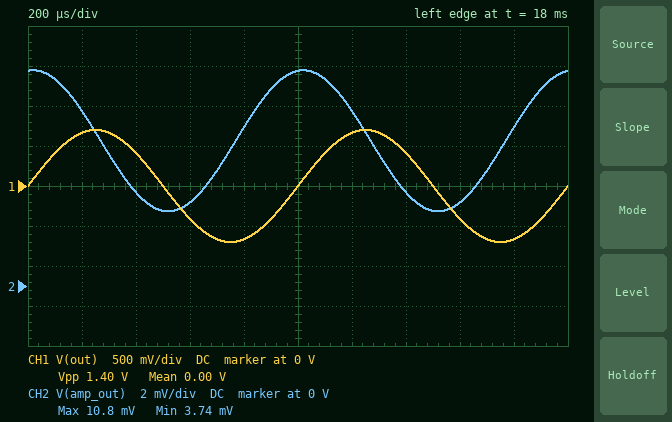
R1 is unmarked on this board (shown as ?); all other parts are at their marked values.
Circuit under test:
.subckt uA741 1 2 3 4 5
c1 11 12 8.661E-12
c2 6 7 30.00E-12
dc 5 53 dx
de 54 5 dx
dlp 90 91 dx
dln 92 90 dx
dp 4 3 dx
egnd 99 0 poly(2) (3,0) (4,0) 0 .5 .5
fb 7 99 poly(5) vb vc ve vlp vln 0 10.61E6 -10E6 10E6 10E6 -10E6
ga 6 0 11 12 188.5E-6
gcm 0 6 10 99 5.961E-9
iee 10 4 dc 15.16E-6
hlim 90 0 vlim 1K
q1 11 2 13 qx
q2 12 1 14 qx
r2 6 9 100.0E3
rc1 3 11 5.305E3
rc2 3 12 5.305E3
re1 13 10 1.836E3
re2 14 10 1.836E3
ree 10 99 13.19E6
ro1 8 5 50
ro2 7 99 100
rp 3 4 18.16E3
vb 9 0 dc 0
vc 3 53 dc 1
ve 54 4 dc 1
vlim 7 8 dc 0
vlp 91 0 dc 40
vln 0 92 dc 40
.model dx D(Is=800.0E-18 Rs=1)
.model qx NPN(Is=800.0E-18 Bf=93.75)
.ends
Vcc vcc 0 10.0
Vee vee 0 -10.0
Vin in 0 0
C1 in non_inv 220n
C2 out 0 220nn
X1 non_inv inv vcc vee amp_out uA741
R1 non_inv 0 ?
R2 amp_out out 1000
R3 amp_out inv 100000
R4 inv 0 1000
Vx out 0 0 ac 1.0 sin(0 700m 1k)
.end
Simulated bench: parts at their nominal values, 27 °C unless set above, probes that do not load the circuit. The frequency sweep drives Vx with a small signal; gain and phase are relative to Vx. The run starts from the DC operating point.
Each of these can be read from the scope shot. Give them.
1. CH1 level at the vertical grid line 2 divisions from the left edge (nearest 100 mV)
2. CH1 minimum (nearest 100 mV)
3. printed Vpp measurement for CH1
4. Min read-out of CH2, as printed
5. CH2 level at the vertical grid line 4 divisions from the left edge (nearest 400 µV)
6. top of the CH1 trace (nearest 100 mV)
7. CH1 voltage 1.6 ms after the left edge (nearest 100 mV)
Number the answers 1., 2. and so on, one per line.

1. 400 mV
2. -700 mV
3. 1.40 V
4. 3.74 mV
5. 8.0 mV
6. 700 mV
7. -400 mV
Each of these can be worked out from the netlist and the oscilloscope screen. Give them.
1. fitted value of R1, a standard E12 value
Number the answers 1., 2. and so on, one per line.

1. 330 Ω
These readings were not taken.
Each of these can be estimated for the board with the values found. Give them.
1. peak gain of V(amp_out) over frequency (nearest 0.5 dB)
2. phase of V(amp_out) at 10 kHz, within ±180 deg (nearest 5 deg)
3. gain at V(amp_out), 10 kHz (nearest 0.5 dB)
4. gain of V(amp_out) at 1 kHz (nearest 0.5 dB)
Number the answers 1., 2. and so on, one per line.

1. -26.5 dB
2. 45 deg
3. -29.0 dB
4. -46.0 dB
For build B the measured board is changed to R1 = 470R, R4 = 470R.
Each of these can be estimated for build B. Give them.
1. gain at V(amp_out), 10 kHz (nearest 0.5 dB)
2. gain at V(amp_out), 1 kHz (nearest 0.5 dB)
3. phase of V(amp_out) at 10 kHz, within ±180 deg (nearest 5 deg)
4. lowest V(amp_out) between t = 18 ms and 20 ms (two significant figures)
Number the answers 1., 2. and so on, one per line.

1. -27.0 dB
2. -39.5 dB
3. 25 deg
4. -3.2 mV
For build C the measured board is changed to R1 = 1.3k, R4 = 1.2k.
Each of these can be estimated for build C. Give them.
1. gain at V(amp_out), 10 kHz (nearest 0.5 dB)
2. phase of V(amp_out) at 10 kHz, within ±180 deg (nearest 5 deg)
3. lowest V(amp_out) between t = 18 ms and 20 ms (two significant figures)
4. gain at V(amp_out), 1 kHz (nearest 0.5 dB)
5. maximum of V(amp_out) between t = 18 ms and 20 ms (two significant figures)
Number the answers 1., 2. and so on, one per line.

1. -30.0 dB
2. 50 deg
3. -2.1 mV
4. -47.5 dB
5. 3.8 mV
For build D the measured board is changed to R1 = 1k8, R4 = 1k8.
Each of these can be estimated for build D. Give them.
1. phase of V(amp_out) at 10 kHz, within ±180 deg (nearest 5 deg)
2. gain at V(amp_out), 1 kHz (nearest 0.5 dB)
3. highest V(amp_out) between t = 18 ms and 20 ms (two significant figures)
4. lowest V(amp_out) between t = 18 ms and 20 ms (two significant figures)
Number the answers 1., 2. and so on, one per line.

1. 60 deg
2. -51.0 dB
3. 2.9 mV
4. -1.0 mV
